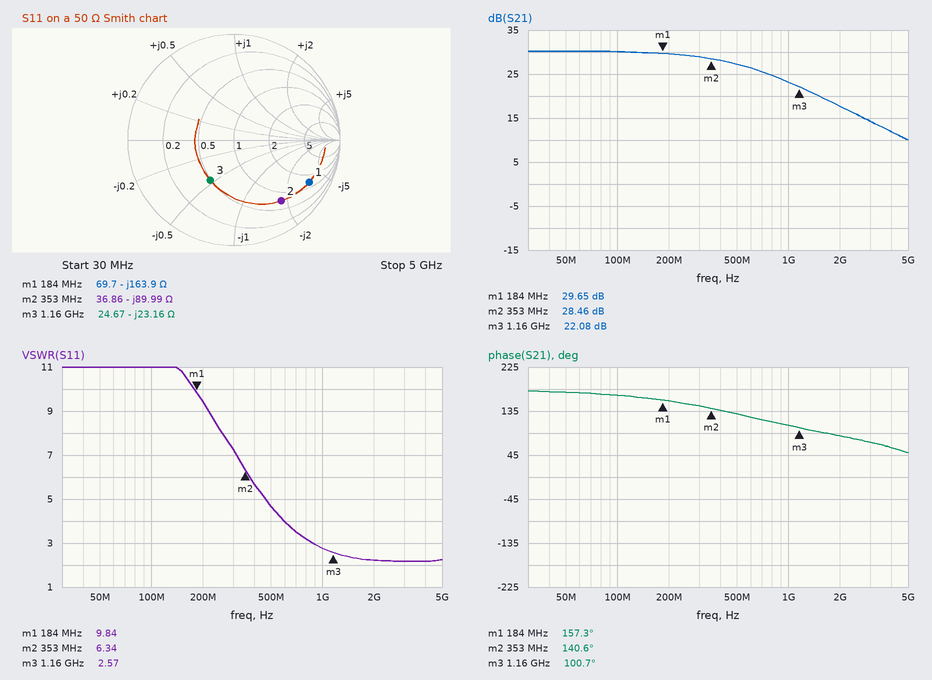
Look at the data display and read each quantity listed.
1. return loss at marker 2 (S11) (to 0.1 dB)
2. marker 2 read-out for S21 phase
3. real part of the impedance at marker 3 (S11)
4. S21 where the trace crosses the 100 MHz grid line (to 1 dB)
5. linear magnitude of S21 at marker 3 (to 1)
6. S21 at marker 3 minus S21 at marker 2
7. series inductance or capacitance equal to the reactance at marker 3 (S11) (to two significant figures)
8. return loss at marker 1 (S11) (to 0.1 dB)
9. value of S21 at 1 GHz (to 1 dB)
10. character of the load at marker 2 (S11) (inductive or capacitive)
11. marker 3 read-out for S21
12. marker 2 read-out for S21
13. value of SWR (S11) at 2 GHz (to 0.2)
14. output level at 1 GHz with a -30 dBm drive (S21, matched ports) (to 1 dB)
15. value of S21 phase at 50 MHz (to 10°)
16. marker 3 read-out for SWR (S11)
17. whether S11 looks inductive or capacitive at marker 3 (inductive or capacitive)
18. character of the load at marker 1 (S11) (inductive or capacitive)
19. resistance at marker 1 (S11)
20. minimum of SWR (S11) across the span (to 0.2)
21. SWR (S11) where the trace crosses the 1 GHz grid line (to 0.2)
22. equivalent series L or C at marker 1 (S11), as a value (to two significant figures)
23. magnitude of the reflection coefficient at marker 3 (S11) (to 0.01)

2.8 dB
140.6°
24.67 Ω
30 dB
13
-6.38 dB
5.9 pF
1.8 dB
23 dB
capacitive
22.08 dB
28.46 dB
2.2
-7 dBm
170°
2.57
capacitive
capacitive
69.7 Ω
2.2
2.8
5.3 pF
0.44
